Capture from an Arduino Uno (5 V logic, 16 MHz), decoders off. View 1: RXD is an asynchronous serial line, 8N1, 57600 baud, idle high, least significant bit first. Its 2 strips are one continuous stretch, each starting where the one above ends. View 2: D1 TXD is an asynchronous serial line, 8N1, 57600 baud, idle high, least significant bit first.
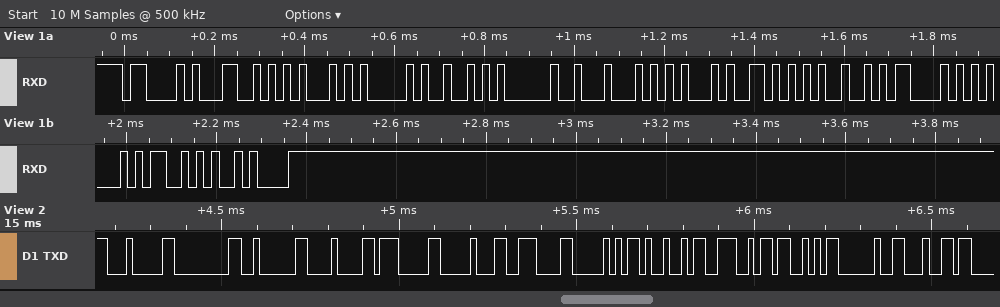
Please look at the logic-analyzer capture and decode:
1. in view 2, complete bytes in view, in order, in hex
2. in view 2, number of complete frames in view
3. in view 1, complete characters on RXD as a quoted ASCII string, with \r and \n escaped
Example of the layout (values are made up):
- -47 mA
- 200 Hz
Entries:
- 04 00 02 08 07 10 0E 50 49 4E 53 20 64
- 13
- "CLEAR DEVICES\n"
